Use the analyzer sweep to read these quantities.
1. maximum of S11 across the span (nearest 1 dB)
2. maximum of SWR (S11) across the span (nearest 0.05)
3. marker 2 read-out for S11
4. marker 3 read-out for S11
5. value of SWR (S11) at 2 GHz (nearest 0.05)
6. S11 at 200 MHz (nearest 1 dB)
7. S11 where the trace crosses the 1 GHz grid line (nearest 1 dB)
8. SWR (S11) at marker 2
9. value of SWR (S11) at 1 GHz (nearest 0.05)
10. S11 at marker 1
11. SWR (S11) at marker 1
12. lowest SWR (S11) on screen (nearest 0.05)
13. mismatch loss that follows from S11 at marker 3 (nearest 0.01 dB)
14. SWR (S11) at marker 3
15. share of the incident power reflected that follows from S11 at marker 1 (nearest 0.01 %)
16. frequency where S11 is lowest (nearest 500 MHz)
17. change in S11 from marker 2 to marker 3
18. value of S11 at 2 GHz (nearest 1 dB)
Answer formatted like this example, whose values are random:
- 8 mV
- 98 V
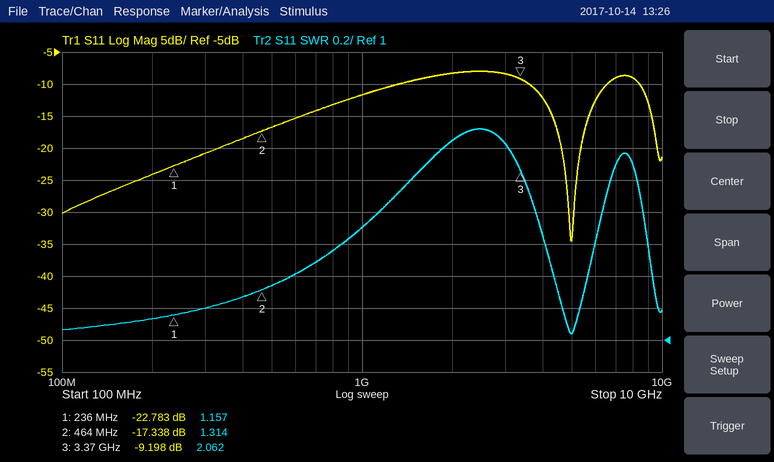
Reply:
- -8 dB
- 2.30
- -17.338 dB
- -9.198 dB
- 2.25
- -24 dB
- -12 dB
- 1.314
- 1.70
- -22.783 dB
- 1.157
- 1.05
- 0.56 dB
- 2.062
- 0.53 %
- 5.0 GHz
- 8.140 dB
- -8 dB
